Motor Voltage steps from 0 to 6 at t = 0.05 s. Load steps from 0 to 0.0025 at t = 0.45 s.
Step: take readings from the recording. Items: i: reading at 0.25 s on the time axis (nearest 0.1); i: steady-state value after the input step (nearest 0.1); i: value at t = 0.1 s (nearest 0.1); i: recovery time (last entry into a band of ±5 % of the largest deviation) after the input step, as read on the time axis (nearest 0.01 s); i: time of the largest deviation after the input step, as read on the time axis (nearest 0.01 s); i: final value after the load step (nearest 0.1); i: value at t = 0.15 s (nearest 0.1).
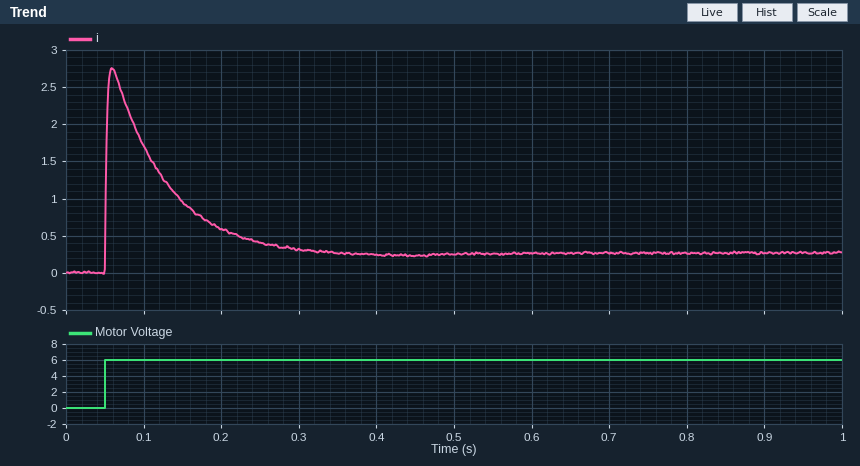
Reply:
0.4
0.2
1.7
0.27 s
0.06 s
0.3
1.0
